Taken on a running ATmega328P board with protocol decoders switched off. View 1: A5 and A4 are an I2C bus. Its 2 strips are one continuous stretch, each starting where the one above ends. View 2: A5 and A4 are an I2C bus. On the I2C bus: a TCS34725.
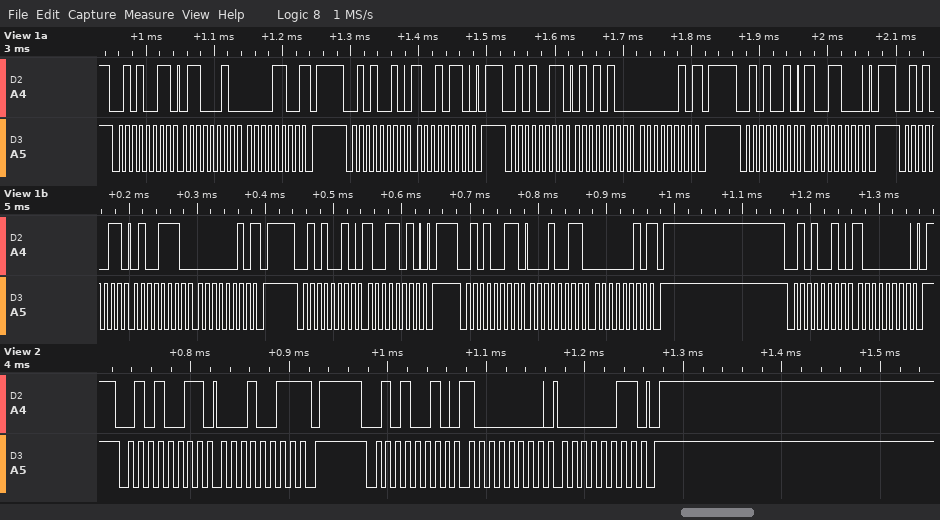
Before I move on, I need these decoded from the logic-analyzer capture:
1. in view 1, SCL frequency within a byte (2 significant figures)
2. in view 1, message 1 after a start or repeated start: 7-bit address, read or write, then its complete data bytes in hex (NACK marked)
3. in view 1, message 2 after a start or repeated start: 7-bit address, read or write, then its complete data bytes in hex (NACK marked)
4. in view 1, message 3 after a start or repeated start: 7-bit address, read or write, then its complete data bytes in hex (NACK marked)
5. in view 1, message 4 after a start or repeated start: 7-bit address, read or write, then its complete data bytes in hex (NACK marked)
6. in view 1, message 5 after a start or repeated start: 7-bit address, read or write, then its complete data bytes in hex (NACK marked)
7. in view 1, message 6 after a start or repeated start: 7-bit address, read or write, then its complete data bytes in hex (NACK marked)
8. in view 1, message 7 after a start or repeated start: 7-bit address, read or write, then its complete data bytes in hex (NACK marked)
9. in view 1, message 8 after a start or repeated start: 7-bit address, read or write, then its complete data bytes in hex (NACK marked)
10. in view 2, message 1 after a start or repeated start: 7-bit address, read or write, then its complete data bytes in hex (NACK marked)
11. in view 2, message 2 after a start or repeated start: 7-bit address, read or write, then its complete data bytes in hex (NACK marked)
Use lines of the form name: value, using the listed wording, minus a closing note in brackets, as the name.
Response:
in view 1, SCL frequency within a byte: 100 kHz
in view 1, message 1 after a start or repeated start: 7-bit address, read or write, then its complete data bytes in hex: 0x29 read: 62 0C NACK
in view 1, message 2 after a start or repeated start: 7-bit address, read or write, then its complete data bytes in hex: 0x29 write: 96
in view 1, message 3 after a start or repeated start: 7-bit address, read or write, then its complete data bytes in hex: 0x29 read: 54 02 NACK
in view 1, message 4 after a start or repeated start: 7-bit address, read or write, then its complete data bytes in hex: 0x29 write: 98
in view 1, message 5 after a start or repeated start: 7-bit address, read or write, then its complete data bytes in hex: 0x29 read: 4E 02 NACK
in view 1, message 6 after a start or repeated start: 7-bit address, read or write, then its complete data bytes in hex: 0x29 write: 9A
in view 1, message 7 after a start or repeated start: 7-bit address, read or write, then its complete data bytes in hex: 0x29 read: 13 02 NACK
in view 1, message 8 after a start or repeated start: 7-bit address, read or write, then its complete data bytes in hex: 0x29 write: 80
in view 2, message 1 after a start or repeated start: 7-bit address, read or write, then its complete data bytes in hex: 0x29 read: 13 NACK
in view 2, message 2 after a start or repeated start: 7-bit address, read or write, then its complete data bytes in hex: 0x29 write: 80 03
